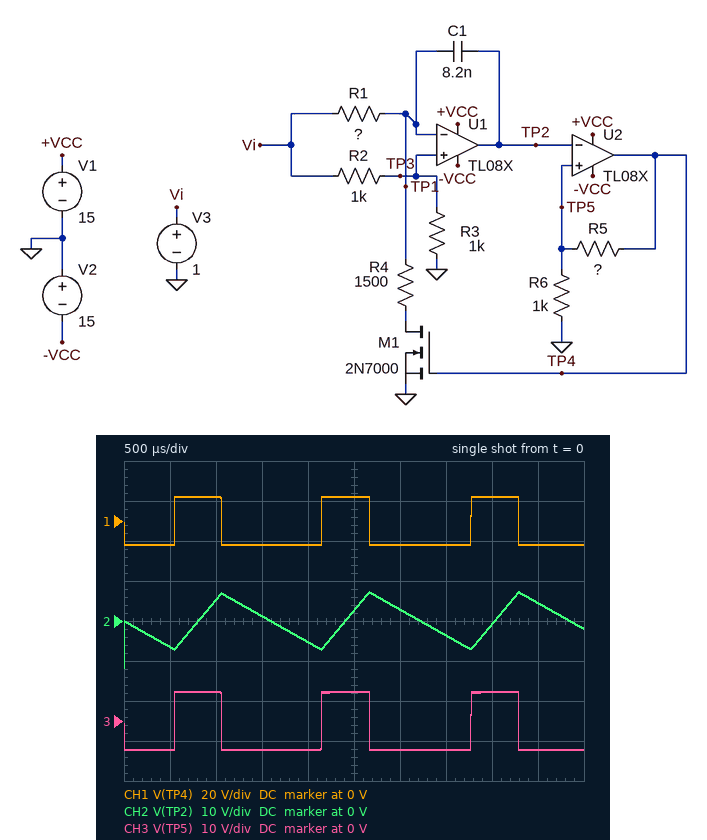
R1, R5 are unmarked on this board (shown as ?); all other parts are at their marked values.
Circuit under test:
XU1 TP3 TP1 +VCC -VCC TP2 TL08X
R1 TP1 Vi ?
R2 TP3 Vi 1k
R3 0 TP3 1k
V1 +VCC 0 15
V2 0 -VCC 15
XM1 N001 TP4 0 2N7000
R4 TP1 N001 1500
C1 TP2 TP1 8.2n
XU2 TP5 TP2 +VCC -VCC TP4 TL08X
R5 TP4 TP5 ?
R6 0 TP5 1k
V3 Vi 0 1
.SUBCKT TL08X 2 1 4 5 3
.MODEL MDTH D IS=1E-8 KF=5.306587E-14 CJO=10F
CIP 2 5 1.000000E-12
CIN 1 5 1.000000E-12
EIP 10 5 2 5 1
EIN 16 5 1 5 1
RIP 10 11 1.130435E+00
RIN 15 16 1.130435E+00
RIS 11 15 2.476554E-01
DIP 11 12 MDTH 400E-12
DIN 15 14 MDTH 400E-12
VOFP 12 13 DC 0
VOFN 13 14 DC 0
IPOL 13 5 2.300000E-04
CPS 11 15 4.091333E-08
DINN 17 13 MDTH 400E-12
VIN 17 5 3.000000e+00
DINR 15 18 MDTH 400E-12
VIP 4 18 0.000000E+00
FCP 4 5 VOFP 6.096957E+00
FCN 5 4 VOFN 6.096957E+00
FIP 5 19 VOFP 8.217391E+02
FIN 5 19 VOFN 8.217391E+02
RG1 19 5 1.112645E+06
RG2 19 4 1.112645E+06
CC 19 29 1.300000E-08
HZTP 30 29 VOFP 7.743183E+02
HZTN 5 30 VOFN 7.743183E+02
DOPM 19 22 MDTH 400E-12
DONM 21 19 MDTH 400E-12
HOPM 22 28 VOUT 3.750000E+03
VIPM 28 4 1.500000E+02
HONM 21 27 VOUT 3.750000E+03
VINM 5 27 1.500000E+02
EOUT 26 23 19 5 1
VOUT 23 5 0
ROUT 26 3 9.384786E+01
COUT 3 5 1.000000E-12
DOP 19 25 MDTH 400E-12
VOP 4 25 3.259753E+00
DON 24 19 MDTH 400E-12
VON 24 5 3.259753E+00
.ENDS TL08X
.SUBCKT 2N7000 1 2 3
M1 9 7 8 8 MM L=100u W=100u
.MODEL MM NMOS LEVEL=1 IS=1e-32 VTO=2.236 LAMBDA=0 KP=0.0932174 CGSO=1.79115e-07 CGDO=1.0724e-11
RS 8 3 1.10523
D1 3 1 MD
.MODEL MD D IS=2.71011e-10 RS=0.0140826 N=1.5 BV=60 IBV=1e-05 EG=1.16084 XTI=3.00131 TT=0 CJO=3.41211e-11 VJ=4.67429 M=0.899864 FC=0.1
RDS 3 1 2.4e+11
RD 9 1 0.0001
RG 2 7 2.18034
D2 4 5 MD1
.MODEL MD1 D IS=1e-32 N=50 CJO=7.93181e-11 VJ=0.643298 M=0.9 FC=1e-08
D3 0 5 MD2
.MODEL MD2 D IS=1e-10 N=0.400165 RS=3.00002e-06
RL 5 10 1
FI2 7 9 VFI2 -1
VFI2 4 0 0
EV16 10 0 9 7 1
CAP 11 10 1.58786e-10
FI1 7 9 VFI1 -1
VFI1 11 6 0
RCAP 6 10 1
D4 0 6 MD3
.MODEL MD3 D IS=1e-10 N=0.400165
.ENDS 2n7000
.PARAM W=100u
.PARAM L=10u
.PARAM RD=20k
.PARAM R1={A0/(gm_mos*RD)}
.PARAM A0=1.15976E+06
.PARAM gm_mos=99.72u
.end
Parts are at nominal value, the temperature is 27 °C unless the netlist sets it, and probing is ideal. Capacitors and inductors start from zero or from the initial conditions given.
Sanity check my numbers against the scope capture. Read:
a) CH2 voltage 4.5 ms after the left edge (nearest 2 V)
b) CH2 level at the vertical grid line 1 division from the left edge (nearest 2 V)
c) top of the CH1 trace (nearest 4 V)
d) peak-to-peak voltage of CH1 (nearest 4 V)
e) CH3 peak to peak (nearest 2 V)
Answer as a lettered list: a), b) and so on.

a) 4 V
b) -6 V
c) 12 V
d) 24 V
e) 14 V
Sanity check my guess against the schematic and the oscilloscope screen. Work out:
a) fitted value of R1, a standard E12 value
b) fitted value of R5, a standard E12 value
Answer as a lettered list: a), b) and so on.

a) 4.7 kΩ
b) 680 Ω
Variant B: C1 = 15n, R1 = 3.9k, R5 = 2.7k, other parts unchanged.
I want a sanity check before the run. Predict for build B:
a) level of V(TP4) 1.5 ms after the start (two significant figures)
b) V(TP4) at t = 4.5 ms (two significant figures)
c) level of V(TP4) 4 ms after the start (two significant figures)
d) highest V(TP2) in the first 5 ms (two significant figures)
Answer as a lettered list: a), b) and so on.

a) -12 V
b) 12 V
c) -12 V
d) 3.4 V
